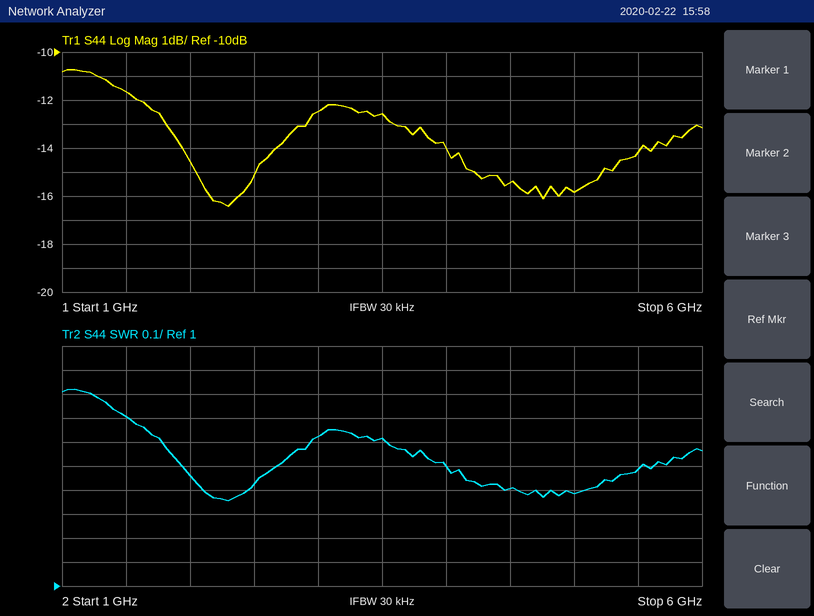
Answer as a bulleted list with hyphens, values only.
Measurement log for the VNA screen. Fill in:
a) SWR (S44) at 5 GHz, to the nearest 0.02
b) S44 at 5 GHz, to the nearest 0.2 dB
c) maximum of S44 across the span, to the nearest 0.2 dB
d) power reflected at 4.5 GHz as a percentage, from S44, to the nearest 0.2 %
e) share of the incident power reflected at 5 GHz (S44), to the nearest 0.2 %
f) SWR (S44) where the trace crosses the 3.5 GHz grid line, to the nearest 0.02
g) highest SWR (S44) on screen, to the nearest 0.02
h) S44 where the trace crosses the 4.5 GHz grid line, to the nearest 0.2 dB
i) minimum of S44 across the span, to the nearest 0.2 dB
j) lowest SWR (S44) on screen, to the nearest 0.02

- 1.38
- -15.8 dB
- -10.8 dB
- 2.8 %
- 2.6 %
- 1.62
- 1.82
- -15.4 dB
- -16.4 dB
- 1.36
